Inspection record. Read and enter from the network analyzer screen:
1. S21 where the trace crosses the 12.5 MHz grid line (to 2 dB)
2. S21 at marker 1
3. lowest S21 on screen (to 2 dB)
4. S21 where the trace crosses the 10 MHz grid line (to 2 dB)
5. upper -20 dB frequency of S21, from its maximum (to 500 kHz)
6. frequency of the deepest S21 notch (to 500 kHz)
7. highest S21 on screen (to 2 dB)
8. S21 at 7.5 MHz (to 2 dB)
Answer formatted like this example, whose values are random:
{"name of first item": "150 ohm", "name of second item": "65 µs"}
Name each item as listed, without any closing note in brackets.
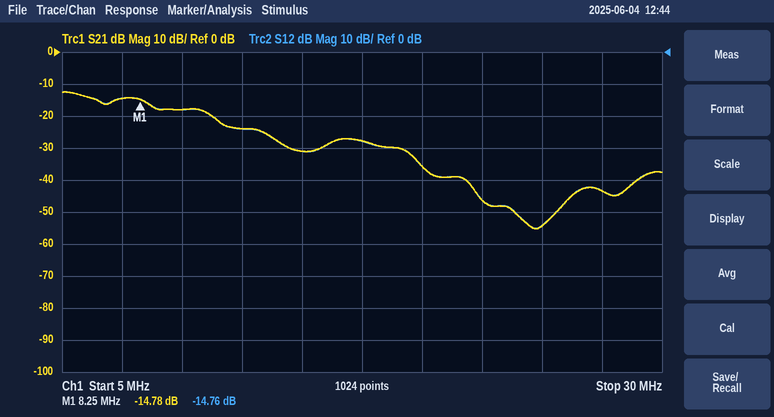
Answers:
{"S21 where the trace crosses the 12.5 MHz grid line": "-24 dB", "S21 at marker 1": "-14.78 dB", "lowest S21 on screen": "-56 dB", "S21 where the trace crosses the 10 MHz grid line": "-18 dB", "upper -20 dB frequency of S21, from its maximum": "19.5 MHz", "frequency of the deepest S21 notch": "24.5 MHz", "highest S21 on screen": "-12 dB", "S21 at 7.5 MHz": "-14 dB"}
